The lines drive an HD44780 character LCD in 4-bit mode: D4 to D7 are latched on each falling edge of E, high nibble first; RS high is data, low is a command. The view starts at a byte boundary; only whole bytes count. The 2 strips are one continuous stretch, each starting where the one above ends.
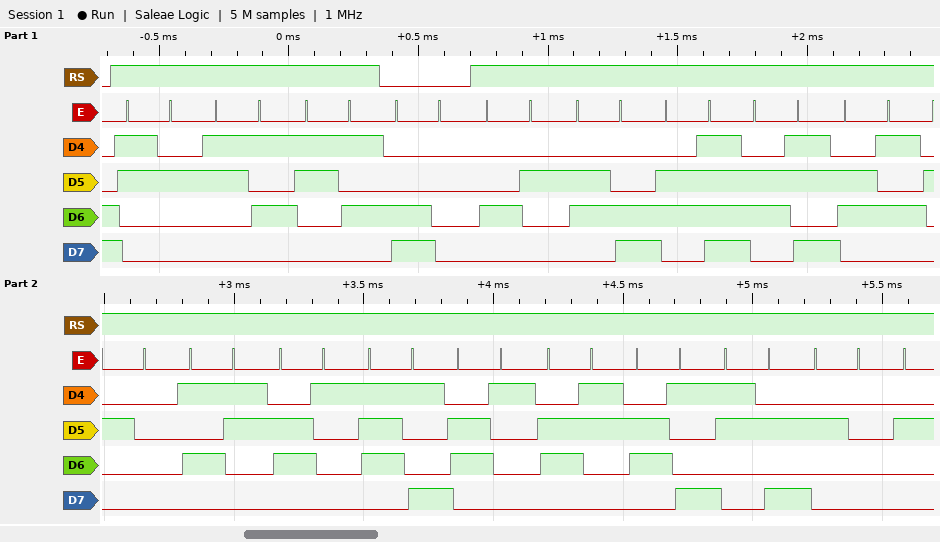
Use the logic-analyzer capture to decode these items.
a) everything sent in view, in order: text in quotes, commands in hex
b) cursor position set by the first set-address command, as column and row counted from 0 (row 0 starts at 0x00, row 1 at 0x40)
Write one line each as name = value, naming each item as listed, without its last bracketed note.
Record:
everything sent in view, in order: text in quotes, commands in hex = "255" 0xC0 "Bloke Sayaci: "
cursor position set by the first set-address command, as column and row counted from 0 = column 0, row 1
